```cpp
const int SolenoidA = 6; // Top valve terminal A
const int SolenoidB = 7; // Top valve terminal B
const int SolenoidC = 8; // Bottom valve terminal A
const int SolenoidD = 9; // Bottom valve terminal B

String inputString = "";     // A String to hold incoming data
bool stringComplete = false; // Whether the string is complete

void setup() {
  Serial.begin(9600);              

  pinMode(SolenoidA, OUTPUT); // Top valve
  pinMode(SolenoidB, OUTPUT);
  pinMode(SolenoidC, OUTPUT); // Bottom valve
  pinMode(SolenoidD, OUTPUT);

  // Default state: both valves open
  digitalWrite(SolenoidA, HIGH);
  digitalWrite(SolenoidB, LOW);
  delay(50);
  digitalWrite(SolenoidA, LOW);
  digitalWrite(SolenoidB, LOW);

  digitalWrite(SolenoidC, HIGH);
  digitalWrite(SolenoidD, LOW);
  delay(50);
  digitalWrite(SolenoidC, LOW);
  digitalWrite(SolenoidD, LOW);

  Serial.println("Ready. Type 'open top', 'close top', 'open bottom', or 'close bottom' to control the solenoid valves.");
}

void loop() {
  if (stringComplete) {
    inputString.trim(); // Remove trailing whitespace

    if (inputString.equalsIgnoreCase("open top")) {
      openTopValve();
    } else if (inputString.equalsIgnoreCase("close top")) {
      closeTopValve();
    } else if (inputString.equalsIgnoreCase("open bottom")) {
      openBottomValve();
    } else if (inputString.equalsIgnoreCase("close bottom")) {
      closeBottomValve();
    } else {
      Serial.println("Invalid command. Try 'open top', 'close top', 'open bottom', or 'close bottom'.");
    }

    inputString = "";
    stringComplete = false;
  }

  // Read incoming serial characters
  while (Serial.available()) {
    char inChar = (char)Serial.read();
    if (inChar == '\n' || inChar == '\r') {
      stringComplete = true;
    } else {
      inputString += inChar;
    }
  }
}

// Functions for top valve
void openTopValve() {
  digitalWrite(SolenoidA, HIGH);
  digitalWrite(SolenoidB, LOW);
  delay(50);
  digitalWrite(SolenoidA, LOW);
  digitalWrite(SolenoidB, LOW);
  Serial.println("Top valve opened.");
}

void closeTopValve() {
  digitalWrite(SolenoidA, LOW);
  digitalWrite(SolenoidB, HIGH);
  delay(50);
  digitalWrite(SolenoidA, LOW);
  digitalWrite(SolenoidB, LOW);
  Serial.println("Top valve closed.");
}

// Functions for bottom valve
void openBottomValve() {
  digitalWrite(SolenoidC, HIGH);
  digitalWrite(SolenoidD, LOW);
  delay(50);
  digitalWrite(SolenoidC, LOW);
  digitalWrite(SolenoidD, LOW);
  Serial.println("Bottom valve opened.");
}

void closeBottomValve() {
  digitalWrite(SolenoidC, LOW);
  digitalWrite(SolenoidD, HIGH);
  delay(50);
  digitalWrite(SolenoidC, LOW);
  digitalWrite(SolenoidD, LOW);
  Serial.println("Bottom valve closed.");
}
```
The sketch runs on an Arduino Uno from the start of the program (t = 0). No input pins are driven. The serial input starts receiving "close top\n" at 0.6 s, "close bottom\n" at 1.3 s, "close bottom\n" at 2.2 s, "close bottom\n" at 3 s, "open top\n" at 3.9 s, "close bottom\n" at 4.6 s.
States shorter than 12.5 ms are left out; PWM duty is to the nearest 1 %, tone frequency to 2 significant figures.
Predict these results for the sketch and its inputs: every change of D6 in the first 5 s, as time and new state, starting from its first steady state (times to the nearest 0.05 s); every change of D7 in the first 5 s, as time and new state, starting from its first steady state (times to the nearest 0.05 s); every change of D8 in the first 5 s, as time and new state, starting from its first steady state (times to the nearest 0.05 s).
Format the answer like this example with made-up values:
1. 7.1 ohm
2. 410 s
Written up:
1. 0 s high; 0.05 s low; 3.9 s high; 3.95 s low
2. 0 s low; 0.6 s high; 0.65 s low
3. 0 s low; 0.05 s high; 0.1 s low
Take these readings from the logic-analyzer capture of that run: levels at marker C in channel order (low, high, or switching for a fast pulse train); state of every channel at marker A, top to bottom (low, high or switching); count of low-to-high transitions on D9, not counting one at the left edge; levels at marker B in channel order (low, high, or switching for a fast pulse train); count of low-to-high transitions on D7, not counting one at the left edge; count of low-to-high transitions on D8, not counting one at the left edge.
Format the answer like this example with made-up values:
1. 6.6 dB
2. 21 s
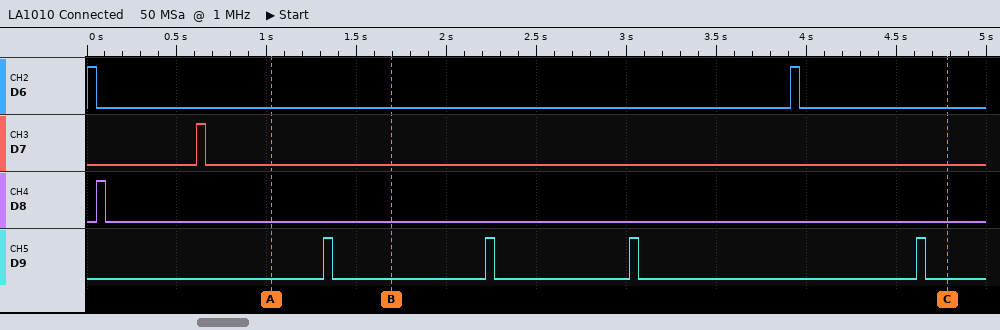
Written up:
1. D6 low, D7 low, D8 low, D9 low
2. D6 low, D7 low, D8 low, D9 low
3. 4
4. D6 low, D7 low, D8 low, D9 low
5. 1
6. 1
